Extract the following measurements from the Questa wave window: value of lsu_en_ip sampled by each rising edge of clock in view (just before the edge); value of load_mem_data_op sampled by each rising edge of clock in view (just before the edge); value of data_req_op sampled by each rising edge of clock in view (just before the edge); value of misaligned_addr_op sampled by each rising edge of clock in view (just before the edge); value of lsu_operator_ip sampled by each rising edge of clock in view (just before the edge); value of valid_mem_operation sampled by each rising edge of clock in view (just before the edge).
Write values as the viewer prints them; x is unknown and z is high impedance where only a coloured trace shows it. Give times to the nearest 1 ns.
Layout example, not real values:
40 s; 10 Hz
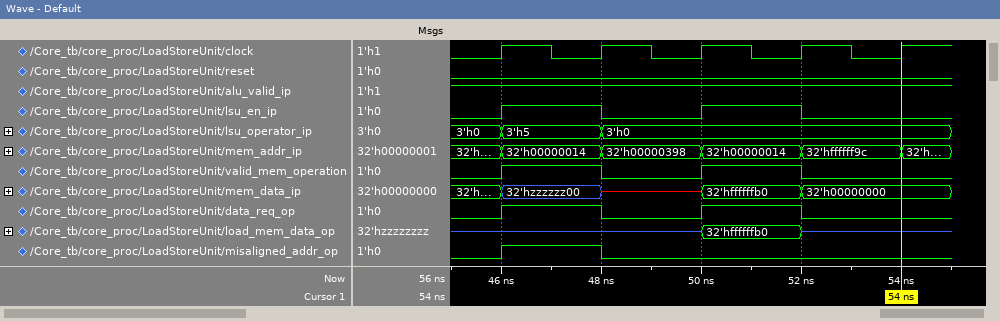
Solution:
0 1 0 1 0; z, z, z, 32'hffffffb0, z; 0 1 0 1 0; 0 1 0 0 0; 3'h0, 3'h5, 3'h0, 3'h0, 3'h0; 0 1 0 1 0
